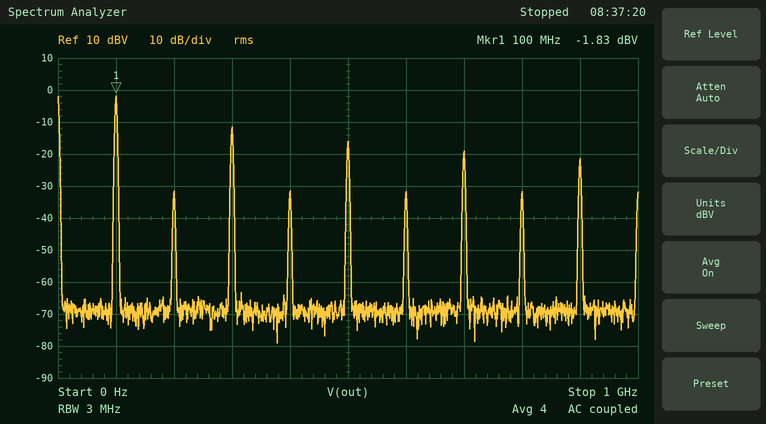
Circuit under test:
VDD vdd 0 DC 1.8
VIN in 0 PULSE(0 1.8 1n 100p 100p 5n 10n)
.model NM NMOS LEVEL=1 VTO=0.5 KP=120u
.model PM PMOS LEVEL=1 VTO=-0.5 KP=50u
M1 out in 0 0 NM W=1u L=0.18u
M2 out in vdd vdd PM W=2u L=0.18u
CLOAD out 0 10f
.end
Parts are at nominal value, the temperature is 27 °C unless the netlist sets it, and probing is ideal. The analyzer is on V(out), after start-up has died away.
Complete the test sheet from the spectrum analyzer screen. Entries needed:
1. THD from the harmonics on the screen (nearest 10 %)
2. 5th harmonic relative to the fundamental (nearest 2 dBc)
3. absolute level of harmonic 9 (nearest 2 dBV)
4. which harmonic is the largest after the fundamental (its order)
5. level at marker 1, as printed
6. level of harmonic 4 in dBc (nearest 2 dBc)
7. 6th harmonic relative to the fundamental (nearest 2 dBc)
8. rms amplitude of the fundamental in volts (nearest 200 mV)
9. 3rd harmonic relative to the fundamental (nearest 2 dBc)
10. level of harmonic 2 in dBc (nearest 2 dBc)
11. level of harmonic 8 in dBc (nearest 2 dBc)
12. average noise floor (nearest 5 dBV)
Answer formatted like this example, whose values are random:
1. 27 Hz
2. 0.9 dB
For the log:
1. 40 %
2. -14 dBc
3. -22 dBV
4. 3
5. -1.83 dBV
6. -30 dBc
7. -30 dBc
8. 800 mV
9. -10 dBc
10. -30 dBc
11. -30 dBc
12. -70 dBV
